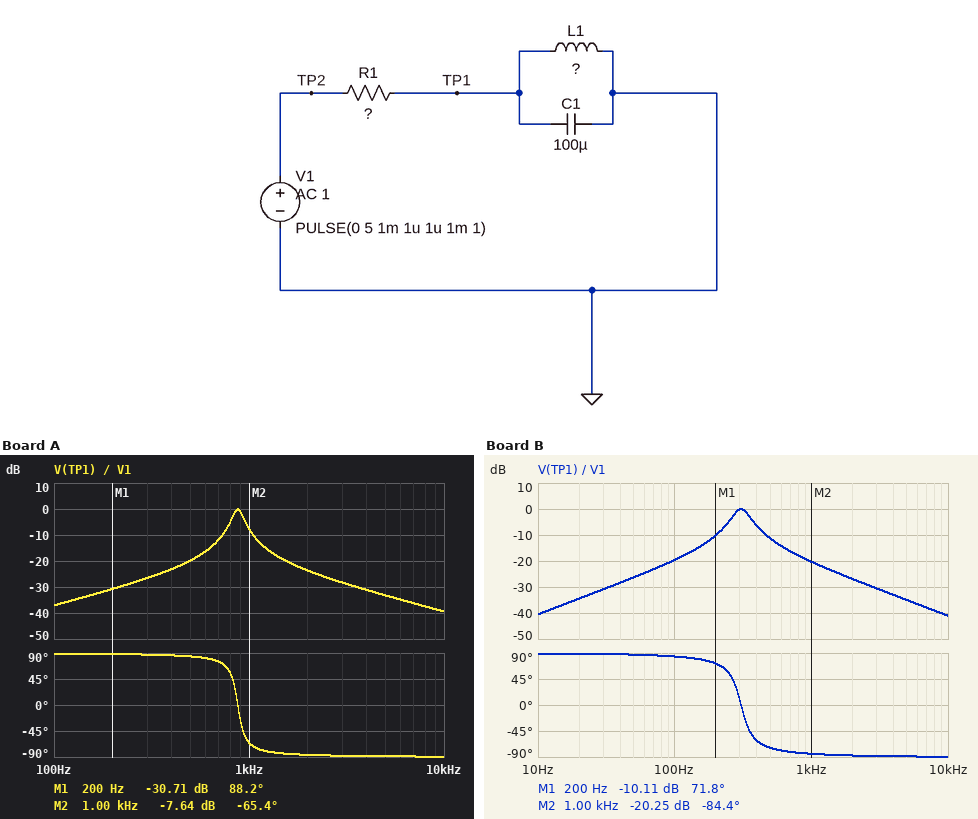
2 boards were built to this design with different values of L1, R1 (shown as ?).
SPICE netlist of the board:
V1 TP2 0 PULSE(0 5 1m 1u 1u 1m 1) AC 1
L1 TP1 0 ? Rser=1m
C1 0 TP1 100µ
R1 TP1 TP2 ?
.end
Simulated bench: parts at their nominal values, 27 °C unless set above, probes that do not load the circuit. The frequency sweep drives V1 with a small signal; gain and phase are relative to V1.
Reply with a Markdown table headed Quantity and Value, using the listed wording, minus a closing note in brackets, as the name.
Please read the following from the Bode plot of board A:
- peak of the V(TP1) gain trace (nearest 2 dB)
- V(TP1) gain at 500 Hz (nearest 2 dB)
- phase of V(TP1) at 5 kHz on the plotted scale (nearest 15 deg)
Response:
| Quantity | Value |
|---|---|
| peak of the V(TP1) gain trace | 0 dB |
| V(TP1) gain at 500 Hz | -20 dB |
| phase of V(TP1) at 5 kHz on the plotted scale | -90 deg |
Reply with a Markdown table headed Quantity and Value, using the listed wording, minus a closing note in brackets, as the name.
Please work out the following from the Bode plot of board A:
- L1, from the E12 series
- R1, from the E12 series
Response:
| Quantity | Value |
|---|---|
| L1, from the E12 series | 330 µH |
| R1, from the E12 series | 15 Ω |
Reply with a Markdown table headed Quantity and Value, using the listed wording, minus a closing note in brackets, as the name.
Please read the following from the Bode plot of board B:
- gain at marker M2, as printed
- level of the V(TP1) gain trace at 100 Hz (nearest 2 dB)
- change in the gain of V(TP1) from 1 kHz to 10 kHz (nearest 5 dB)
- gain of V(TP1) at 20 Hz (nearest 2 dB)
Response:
| Quantity | Value |
|---|---|
| gain at marker M2, as printed | -20.25 dB |
| level of the V(TP1) gain trace at 100 Hz | -20 dB |
| change in the gain of V(TP1) from 1 kHz to 10 kHz | -20 dB |
| gain of V(TP1) at 20 Hz | -34 dB |
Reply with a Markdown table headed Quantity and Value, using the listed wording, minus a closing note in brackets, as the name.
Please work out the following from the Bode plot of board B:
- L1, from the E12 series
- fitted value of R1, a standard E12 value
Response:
| Quantity | Value |
|---|---|
| L1, from the E12 series | 2.7 mH |
| fitted value of R1, a standard E12 value | 18 Ω |
